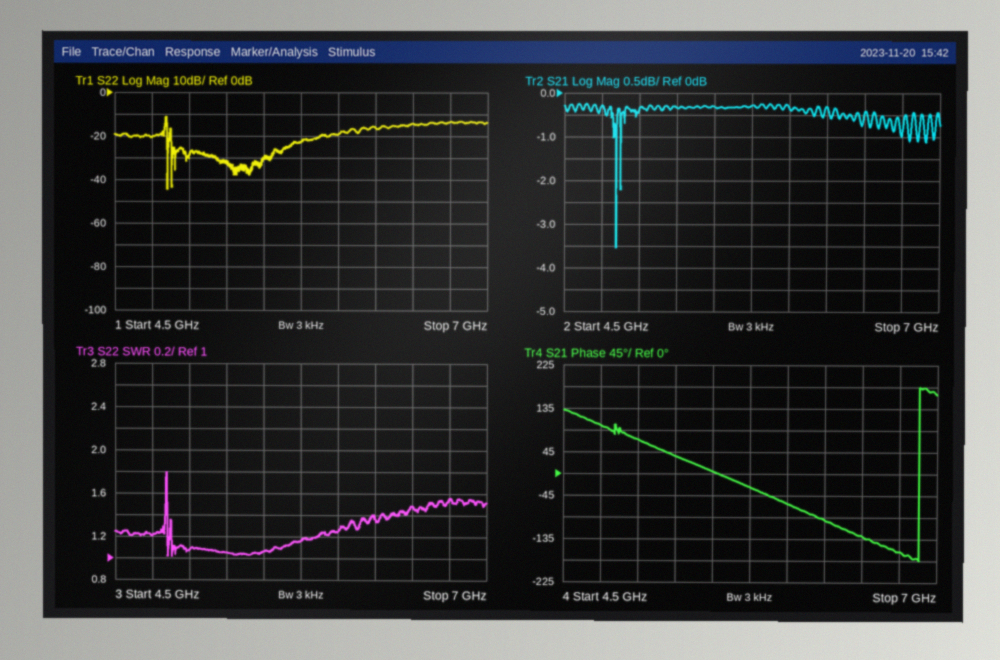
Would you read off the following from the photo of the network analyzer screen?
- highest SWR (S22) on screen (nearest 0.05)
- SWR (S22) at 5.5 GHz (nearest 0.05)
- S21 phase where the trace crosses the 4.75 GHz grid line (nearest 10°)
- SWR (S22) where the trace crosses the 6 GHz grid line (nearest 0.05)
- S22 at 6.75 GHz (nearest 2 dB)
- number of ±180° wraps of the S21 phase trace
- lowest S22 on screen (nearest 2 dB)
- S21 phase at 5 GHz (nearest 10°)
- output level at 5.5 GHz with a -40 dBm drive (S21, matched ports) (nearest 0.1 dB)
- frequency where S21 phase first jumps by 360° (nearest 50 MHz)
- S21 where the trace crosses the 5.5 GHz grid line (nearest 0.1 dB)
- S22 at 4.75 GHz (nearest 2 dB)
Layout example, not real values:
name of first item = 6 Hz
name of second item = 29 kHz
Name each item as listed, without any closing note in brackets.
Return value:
highest SWR (S22) on screen = 1.80
SWR (S22) at 5.5 GHz = 1.05
S21 phase where the trace crosses the 4.75 GHz grid line = 100°
SWR (S22) where the trace crosses the 6 GHz grid line = 1.25
S22 at 6.75 GHz = -14 dB
number of ±180° wraps of the S21 phase trace = 1
lowest S22 on screen = -44 dB
S21 phase at 5 GHz = 70°
output level at 5.5 GHz with a -40 dBm drive (S21, matched ports) = -40.3 dBm
frequency where S21 phase first jumps by 360° = 6.90 GHz
S21 where the trace crosses the 5.5 GHz grid line = -0.3 dB
S22 at 4.75 GHz = -20 dB
